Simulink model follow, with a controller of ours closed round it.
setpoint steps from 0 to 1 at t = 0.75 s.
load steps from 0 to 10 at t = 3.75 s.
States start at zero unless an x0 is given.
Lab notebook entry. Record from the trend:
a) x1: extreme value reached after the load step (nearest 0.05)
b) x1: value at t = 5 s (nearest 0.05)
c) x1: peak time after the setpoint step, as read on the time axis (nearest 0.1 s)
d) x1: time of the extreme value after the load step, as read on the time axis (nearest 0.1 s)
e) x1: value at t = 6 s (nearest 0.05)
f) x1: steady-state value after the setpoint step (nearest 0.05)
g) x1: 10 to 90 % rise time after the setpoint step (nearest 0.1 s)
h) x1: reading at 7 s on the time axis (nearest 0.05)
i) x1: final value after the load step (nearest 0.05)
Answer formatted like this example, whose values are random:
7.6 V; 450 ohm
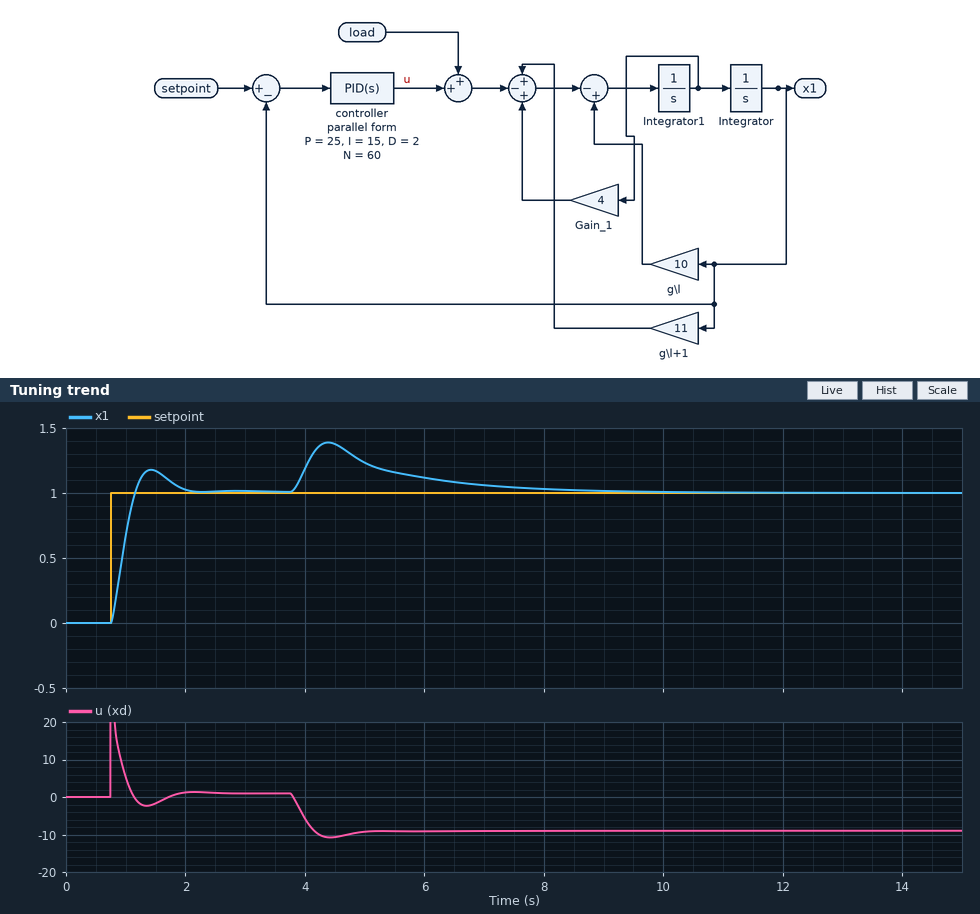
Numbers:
1.40; 1.25; 1.4 s; 4.4 s; 1.10; 1.00; 0.3 s; 1.05; 1.00
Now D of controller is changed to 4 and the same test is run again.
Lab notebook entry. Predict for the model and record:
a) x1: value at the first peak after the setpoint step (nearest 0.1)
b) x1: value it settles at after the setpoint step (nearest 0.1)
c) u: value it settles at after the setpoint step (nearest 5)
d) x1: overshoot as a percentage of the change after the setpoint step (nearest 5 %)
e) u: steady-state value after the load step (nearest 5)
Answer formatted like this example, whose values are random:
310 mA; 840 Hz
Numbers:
1.1; 1.0; 0; 10 %; -10
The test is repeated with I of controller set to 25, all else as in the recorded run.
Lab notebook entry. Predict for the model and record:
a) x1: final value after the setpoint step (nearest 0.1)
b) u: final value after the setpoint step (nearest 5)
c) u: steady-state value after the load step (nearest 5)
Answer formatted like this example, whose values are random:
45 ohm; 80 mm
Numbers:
1.0; 0; -10
